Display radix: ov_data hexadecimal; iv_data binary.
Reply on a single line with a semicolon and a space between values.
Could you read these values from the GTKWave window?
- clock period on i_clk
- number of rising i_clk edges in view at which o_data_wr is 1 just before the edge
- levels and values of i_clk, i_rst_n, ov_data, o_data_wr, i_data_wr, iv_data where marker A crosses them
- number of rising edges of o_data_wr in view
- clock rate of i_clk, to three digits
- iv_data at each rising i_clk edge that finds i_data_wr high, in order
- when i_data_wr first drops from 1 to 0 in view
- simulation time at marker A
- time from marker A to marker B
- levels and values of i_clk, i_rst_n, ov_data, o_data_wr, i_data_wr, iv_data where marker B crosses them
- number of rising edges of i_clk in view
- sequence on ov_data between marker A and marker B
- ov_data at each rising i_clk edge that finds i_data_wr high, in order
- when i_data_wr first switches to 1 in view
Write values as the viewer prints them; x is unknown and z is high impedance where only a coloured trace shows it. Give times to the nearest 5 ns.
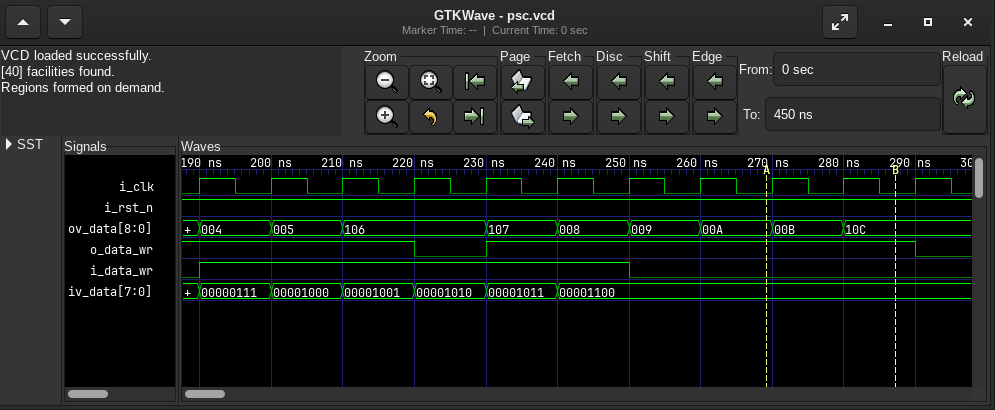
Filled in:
10 ns; 10; i_clk=0, i_rst_n=1, ov_data=00A, o_data_wr=1, i_data_wr=0, iv_data=00001100; 1; 100 MHz; 00000111, 00001000, 00001001, 00001010, 00001011, 00001100; 250 ns; 270 ns; 20 ns; i_clk=0, i_rst_n=1, ov_data=10C, o_data_wr=1, i_data_wr=0, iv_data=00001100; 11; 00A, 00B, 10C; 004, 005, 106, 106, 107, 008; 190 ns
